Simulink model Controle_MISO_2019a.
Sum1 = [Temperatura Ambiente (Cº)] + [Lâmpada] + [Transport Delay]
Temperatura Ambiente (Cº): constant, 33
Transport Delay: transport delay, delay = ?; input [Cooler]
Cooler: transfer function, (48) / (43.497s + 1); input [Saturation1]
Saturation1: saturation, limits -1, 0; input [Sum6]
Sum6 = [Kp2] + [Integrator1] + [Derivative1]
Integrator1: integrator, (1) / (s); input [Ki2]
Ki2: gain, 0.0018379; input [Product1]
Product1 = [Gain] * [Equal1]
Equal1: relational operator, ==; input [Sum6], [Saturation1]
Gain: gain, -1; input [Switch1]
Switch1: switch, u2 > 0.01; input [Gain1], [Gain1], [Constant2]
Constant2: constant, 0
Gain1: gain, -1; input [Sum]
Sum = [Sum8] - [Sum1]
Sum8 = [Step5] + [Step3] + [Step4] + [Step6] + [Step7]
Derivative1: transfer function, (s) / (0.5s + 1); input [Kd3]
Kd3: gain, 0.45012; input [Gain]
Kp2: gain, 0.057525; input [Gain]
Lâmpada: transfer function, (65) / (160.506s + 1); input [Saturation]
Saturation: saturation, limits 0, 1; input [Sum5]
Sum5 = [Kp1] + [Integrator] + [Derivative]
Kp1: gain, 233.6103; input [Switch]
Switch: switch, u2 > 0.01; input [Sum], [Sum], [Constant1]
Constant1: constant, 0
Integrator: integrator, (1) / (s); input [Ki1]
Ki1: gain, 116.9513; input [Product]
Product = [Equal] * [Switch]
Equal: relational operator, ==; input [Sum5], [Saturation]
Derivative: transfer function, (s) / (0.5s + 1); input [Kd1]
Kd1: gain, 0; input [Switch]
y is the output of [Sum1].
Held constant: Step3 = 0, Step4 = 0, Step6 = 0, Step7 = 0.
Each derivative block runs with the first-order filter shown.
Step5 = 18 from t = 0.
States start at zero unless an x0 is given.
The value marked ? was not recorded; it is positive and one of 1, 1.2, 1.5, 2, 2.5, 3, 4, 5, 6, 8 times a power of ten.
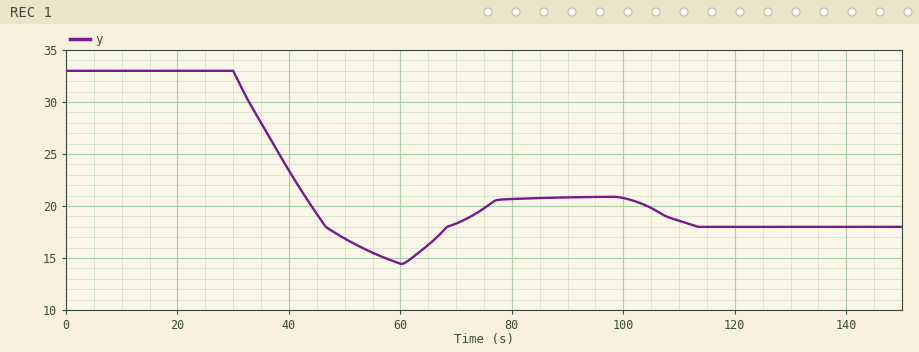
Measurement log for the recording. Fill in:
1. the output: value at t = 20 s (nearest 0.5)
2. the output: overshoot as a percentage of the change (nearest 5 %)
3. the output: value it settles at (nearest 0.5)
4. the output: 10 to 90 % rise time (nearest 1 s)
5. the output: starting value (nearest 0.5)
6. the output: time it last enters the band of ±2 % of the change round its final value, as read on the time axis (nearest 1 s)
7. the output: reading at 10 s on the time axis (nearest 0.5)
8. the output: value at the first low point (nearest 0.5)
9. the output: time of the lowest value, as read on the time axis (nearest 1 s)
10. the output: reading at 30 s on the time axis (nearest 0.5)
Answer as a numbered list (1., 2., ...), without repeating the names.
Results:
1. 33.0
2. 25 %
3. 18.0
4. 13 s
5. 33.0
6. 112 s
7. 33.0
8. 14.5
9. 60 s
10. 33.0
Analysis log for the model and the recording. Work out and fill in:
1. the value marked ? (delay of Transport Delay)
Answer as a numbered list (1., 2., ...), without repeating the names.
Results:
1. 30
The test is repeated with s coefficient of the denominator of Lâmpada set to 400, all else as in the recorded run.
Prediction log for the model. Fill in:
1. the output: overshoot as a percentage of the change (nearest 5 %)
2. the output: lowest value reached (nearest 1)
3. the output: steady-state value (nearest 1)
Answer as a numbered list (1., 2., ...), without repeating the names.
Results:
1. 45 %
2. 11
3. 18
